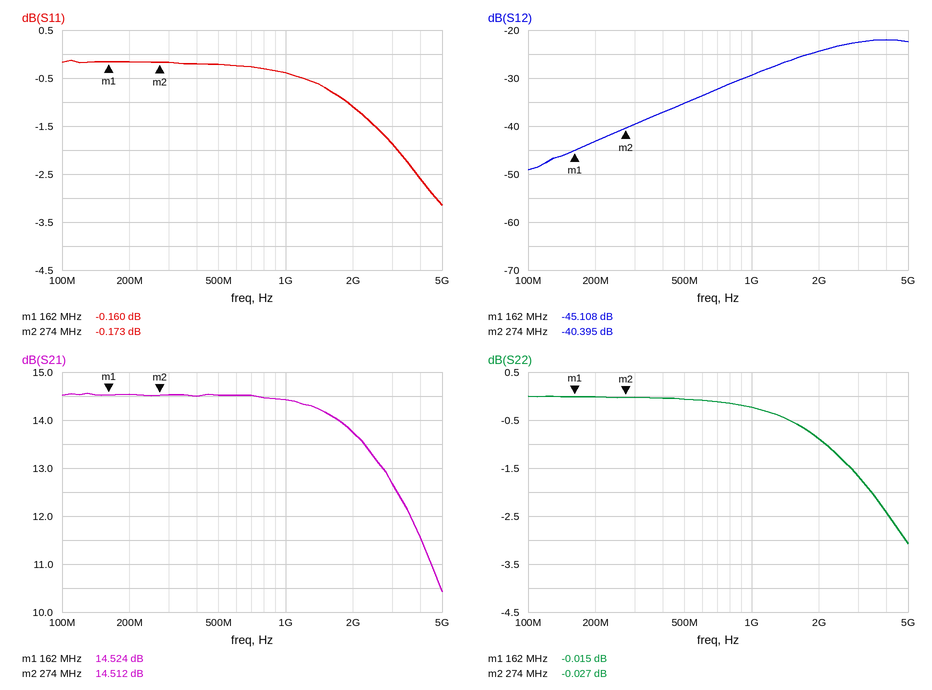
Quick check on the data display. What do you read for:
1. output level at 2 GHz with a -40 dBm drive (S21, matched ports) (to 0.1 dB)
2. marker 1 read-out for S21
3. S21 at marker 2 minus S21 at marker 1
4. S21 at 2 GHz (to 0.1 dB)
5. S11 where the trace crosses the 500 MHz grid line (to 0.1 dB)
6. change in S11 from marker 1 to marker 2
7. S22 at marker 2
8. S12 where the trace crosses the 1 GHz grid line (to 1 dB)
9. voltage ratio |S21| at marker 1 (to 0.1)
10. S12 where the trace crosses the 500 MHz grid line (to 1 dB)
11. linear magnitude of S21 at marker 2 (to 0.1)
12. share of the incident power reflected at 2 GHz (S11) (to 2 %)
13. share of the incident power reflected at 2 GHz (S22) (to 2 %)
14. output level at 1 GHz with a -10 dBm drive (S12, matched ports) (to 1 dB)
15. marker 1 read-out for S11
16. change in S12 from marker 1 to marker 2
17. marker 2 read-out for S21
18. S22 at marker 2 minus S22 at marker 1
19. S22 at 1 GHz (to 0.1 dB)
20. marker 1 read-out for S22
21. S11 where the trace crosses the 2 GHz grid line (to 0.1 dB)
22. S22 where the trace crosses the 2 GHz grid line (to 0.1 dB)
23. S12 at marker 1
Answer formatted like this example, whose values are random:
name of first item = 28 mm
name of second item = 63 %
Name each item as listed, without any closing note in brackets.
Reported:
output level at 2 GHz with a -40 dBm drive (S21, matched ports) = -26.3 dBm
marker 1 read-out for S21 = 14.524 dB
S21 at marker 2 minus S21 at marker 1 = -0.012 dB
S21 at 2 GHz = 13.7 dB
S11 where the trace crosses the 500 MHz grid line = -0.2 dB
change in S11 from marker 1 to marker 2 = -0.013 dB
S22 at marker 2 = -0.027 dB
S12 where the trace crosses the 1 GHz grid line = -29 dB
voltage ratio |S21| at marker 1 = 5.3
S12 where the trace crosses the 500 MHz grid line = -35 dB
linear magnitude of S21 at marker 2 = 5.3
share of the incident power reflected at 2 GHz (S11) = 78 %
share of the incident power reflected at 2 GHz (S22) = 82 %
output level at 1 GHz with a -10 dBm drive (S12, matched ports) = -39 dBm
marker 1 read-out for S11 = -0.160 dB
change in S12 from marker 1 to marker 2 = 4.713 dB
marker 2 read-out for S21 = 14.512 dB
S22 at marker 2 minus S22 at marker 1 = -0.012 dB
S22 at 1 GHz = -0.2 dB
marker 1 read-out for S22 = -0.015 dB
S11 where the trace crosses the 2 GHz grid line = -1.1 dB
S22 where the trace crosses the 2 GHz grid line = -0.9 dB
S12 at marker 1 = -45.108 dB
